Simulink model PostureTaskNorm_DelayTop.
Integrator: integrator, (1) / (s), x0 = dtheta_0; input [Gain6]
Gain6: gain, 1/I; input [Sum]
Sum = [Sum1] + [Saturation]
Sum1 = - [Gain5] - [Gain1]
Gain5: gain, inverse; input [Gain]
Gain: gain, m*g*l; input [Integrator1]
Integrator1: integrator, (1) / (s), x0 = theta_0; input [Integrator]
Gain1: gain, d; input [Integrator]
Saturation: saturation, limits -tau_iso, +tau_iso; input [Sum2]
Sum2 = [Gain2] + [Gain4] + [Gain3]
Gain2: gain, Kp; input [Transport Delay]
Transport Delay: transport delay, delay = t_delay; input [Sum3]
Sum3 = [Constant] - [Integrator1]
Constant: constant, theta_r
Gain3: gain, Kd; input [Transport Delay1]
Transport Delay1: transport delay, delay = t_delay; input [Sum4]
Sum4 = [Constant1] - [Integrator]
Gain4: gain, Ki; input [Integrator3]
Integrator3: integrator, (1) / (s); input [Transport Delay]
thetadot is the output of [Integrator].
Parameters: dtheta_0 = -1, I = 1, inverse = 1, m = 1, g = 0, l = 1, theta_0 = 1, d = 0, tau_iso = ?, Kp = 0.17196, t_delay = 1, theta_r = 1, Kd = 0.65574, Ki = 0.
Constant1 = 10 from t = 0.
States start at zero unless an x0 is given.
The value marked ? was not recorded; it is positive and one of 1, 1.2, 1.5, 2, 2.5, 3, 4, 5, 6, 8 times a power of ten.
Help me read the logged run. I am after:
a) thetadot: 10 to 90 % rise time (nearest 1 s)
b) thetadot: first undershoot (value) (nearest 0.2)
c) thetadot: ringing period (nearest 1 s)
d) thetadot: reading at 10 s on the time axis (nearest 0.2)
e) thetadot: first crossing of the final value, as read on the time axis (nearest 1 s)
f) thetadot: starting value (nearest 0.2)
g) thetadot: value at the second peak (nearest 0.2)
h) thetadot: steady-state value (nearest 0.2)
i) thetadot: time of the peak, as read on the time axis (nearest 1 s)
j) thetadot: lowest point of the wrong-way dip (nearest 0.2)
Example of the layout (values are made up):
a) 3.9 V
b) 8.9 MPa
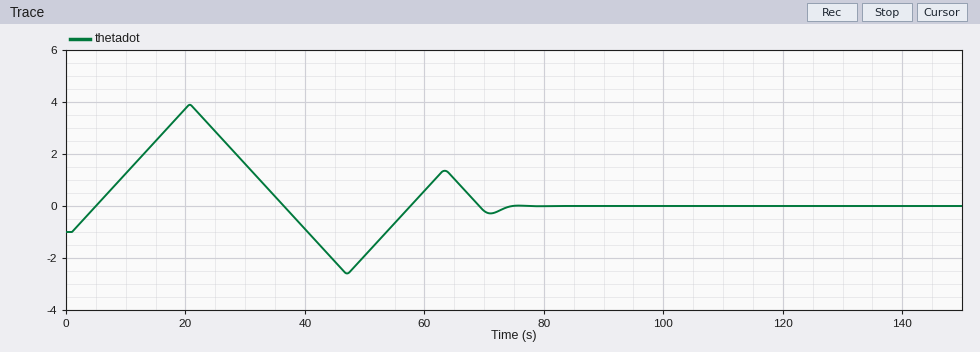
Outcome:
a) 3 s
b) -2.6
c) 43 s
d) 1.2
e) 5 s
f) -1.0
g) 1.4
h) 0.0
i) 21 s
j) -2.6
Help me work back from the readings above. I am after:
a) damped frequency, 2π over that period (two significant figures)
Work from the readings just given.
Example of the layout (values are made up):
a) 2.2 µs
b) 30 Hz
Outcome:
a) 0.15 rad/s
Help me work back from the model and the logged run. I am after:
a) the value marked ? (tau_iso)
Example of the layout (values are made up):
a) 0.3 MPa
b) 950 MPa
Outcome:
a) 0.25
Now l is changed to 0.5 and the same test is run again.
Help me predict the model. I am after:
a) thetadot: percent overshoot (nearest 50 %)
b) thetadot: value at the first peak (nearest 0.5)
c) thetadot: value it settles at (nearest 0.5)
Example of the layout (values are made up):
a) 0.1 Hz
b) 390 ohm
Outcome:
a) 400 %
b) 4.0
c) 0.0
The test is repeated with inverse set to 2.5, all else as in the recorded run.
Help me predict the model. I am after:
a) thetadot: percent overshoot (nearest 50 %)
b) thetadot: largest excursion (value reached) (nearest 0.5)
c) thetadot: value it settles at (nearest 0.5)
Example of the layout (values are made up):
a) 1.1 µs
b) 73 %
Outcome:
a) 400 %
b) 4.0
c) 0.0
